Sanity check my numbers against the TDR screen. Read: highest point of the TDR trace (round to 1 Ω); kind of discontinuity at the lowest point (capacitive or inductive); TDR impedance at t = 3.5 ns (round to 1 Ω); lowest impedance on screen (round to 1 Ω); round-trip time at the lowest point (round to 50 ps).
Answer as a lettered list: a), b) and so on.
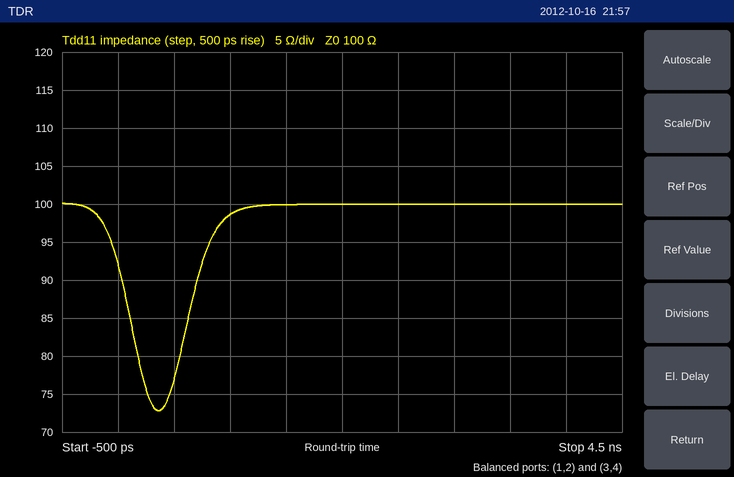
a) 100 Ω
b) capacitive
c) 100 Ω
d) 73 Ω
e) 350 ps
